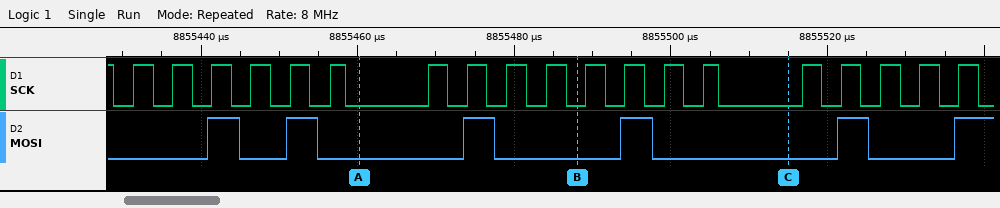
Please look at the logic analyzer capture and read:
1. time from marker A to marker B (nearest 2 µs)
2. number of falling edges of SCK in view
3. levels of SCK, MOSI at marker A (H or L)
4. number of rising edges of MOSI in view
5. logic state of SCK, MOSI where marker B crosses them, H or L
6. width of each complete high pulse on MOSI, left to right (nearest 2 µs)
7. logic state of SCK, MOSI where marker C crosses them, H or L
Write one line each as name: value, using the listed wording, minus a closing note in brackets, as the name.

time from marker A to marker B: 28 µs
number of falling edges of SCK in view: 20
levels of SCK, MOSI at marker A: SCK=L, MOSI=L
number of rising edges of MOSI in view: 6
logic state of SCK, MOSI where marker B crosses them, H or L: SCK=L, MOSI=L
width of each complete high pulse on MOSI, left to right: 4 µs, 4 µs, 4 µs, 4 µs, 4 µs
logic state of SCK, MOSI where marker C crosses them, H or L: SCK=L, MOSI=L
